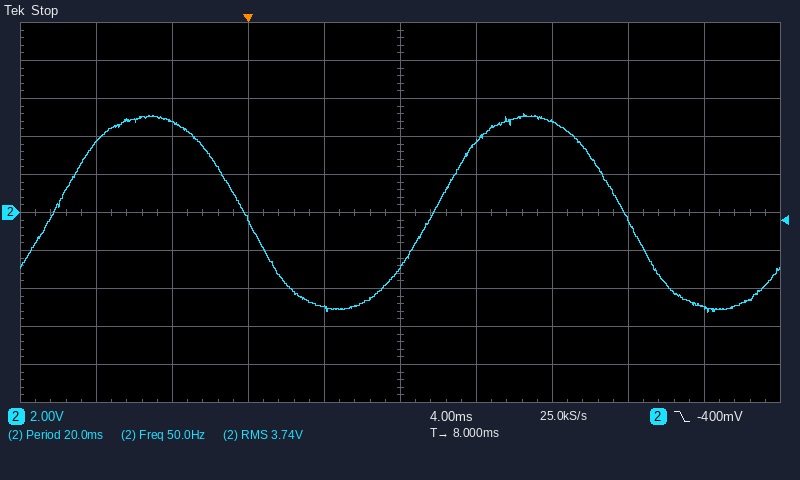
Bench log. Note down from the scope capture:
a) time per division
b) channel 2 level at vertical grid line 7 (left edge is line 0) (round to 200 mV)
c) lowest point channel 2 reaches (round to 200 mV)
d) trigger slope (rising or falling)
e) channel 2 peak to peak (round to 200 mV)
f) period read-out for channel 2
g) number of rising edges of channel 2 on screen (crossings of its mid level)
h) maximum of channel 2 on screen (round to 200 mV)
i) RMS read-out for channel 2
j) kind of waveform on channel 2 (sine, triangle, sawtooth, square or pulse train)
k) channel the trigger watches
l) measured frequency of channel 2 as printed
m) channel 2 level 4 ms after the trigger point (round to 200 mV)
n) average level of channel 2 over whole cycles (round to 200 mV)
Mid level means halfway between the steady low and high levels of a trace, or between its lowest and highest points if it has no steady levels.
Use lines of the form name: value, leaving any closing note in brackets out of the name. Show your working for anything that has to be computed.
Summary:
time per division: 4 ms
channel 2 level at vertical grid line 7 (left edge is line 0): 4.8 V
lowest point channel 2 reaches: -5.2 V
trigger slope: falling
channel 2 peak to peak: 5.2 V − (-5.2 V) = 10.4 V
period read-out for channel 2: 20.0 ms
number of rising edges of channel 2 on screen: 2
maximum of channel 2 on screen: 5.2 V
RMS read-out for channel 2: 3.74 V
kind of waveform on channel 2: sine
channel the trigger watches: channel 2
measured frequency of channel 2 as printed: 50.0 Hz
channel 2 level 4 ms after the trigger point: -5.0 V
average level of channel 2 over whole cycles: (5.2 V + (-5.2 V)) / 2 ≈ 0.0 V
